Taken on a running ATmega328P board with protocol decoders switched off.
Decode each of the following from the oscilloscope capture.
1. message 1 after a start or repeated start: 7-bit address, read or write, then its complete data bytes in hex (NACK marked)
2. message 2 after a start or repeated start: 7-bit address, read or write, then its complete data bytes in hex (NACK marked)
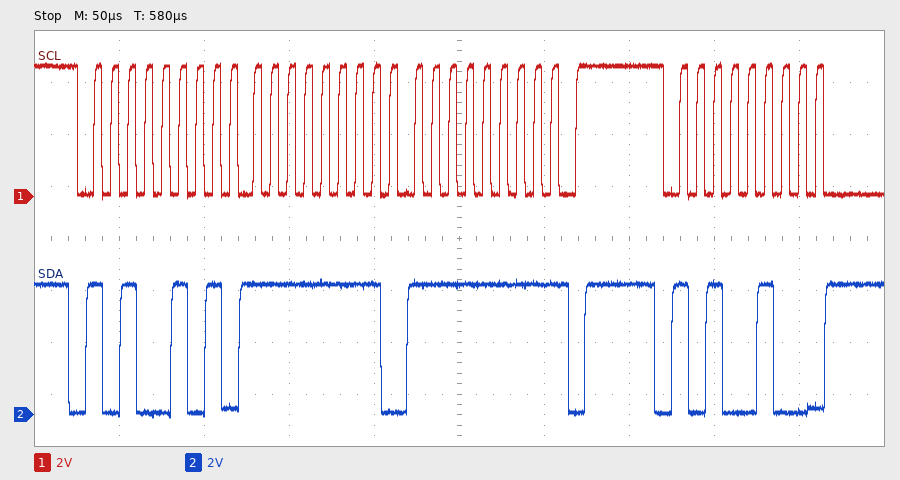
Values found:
0x52 read: FF FF NACK
0x52 write
